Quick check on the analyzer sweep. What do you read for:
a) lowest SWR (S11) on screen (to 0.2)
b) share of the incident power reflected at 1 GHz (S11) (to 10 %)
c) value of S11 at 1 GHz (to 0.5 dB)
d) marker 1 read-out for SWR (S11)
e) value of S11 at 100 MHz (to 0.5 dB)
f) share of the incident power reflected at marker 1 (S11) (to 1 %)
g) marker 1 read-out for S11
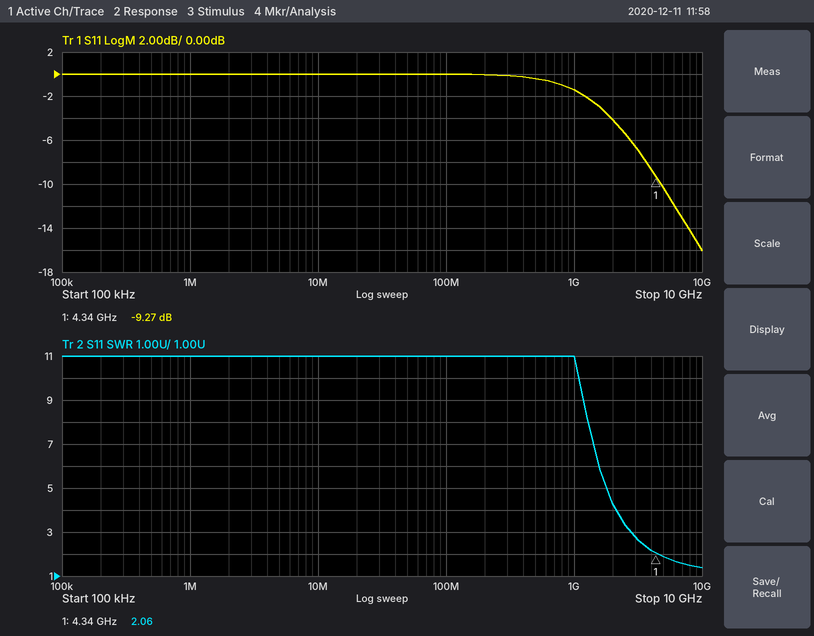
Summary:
1.4
70 %
-1.5 dB
2.06
0.0 dB
12 %
-9.27 dB
